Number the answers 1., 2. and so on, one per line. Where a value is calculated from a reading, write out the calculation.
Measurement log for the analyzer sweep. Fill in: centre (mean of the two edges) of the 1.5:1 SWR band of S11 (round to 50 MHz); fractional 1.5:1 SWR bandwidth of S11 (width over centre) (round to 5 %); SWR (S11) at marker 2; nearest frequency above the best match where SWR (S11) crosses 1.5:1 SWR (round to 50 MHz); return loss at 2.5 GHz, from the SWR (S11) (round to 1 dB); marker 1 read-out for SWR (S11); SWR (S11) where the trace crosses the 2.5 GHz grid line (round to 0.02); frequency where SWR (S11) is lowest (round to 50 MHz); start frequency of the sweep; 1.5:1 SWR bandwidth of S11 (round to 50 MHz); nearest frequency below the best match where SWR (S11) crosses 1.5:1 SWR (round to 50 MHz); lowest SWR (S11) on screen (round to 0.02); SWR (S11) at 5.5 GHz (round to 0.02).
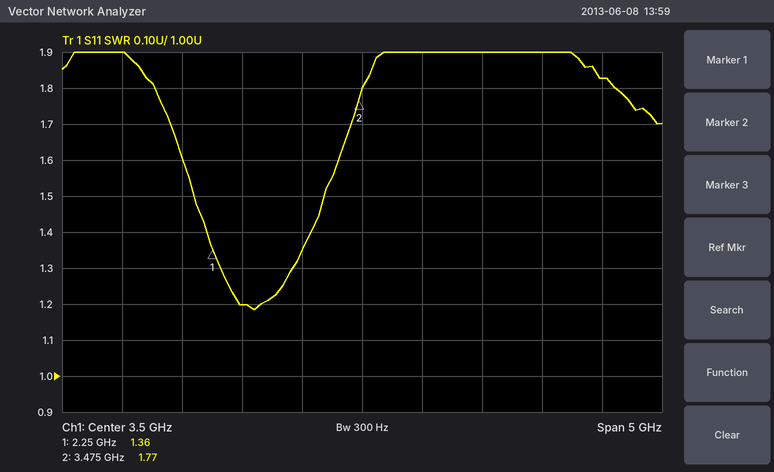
1. 2.65 GHz
2. 1.1 GHz / 2.65 GHz ≈ 41.5 %, so 40 % to the nearest 5 %
3. 1.77
4. 3.20 GHz
5. −20 log10((1.2 − 1)/(1.2 + 1)) ≈ 21 dB
6. 1.36
7. 1.20
8. 2.60 GHz
9. 1 GHz
10. 3.20 GHz − 2.10 GHz = 1.10 GHz
11. 2.10 GHz
12. 1.18
13. 1.82
